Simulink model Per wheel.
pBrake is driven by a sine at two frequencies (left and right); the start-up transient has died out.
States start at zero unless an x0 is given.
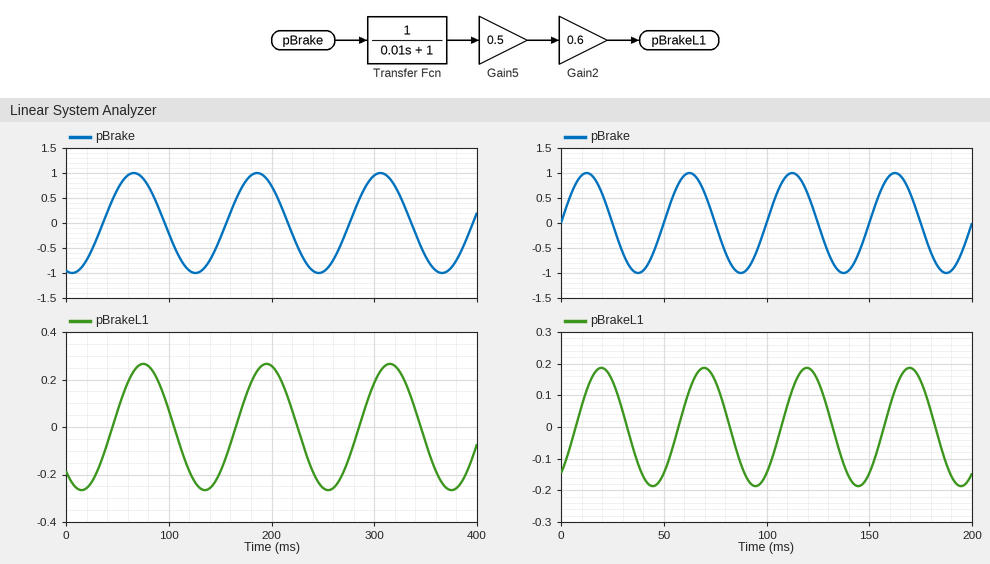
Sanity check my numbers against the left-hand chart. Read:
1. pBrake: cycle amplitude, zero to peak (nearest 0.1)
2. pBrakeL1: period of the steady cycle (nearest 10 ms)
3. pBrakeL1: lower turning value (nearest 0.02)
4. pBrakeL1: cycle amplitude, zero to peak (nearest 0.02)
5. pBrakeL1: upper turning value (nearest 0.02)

1.0
120 ms
-0.26
0.26
0.26
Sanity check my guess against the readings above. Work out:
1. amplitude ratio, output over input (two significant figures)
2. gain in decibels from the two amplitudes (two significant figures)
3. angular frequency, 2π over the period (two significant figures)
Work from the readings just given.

0.26
-12 dB
0.052 rad/ms
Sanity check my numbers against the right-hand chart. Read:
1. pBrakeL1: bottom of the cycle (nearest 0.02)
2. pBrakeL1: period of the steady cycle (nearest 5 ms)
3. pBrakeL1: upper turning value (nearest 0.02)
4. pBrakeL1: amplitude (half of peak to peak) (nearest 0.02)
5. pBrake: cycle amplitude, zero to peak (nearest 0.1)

-0.18
50 ms
0.18
0.18
1.0
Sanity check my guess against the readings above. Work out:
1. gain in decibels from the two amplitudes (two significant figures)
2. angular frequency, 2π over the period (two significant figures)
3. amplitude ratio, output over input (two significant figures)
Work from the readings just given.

-15 dB
0.13 rad/ms
0.18
